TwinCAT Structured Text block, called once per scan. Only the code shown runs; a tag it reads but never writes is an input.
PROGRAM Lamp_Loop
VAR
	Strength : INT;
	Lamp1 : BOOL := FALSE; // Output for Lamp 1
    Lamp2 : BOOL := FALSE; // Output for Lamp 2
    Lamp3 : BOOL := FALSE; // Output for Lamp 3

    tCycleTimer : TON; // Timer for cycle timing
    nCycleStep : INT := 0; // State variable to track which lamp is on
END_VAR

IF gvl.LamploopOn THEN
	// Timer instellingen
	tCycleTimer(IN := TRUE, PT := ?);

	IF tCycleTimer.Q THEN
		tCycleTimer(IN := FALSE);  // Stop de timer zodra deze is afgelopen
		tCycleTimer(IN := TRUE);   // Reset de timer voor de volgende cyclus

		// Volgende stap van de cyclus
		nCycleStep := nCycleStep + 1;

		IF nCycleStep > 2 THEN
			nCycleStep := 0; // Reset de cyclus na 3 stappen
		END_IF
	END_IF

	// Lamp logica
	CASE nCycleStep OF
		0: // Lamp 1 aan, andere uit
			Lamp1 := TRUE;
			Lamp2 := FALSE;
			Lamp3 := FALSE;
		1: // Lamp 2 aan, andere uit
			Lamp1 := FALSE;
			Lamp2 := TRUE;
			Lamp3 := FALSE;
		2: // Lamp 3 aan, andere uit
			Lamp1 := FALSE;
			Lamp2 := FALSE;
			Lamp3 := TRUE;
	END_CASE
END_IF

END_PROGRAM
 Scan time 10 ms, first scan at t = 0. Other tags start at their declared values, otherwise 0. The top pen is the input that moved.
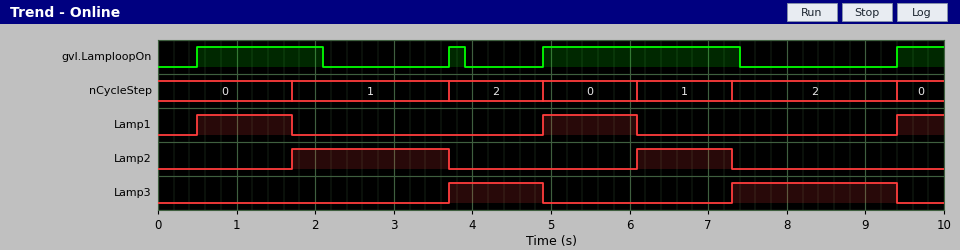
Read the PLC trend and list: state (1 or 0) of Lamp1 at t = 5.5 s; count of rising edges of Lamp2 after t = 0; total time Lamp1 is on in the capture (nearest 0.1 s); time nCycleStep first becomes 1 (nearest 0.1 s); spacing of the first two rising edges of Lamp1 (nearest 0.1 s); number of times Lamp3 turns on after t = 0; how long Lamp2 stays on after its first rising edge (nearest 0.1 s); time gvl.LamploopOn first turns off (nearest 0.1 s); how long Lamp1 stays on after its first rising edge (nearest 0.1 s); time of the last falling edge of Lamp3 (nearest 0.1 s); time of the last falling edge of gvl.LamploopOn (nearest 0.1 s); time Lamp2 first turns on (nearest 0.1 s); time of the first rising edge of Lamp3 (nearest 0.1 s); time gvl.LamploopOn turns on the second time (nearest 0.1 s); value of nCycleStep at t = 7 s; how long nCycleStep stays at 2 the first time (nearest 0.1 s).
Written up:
1
2
3.0 s
1.7 s
4.4 s
2
2.0 s
2.1 s
1.2 s
9.4 s
7.4 s
1.7 s
3.7 s
3.7 s
1
1.2 s
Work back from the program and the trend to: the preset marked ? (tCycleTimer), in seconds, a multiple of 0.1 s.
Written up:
1.2 s
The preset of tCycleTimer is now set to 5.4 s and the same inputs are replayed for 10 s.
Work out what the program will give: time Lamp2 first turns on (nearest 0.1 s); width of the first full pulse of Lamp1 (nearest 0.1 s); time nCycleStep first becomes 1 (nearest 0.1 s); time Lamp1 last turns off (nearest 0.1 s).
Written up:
5.9 s
5.4 s
5.9 s
5.9 s
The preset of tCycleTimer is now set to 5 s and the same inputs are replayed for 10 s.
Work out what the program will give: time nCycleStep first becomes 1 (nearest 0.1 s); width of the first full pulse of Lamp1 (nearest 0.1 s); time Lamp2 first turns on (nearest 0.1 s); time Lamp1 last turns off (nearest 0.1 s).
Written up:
5.5 s
5.0 s
5.5 s
5.5 s
